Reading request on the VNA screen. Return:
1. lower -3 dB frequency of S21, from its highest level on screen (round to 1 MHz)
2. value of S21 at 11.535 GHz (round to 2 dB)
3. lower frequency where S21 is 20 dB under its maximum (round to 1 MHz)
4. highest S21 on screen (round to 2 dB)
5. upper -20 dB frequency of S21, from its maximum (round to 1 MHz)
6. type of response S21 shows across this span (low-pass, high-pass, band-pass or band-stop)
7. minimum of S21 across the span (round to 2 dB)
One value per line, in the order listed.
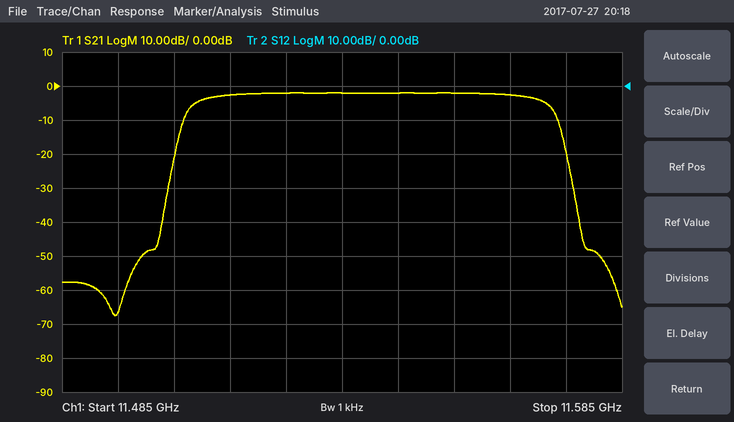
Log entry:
11.509 GHz
-2 dB
11.505 GHz
-2 dB
11.575 GHz
band-pass
-68 dB
